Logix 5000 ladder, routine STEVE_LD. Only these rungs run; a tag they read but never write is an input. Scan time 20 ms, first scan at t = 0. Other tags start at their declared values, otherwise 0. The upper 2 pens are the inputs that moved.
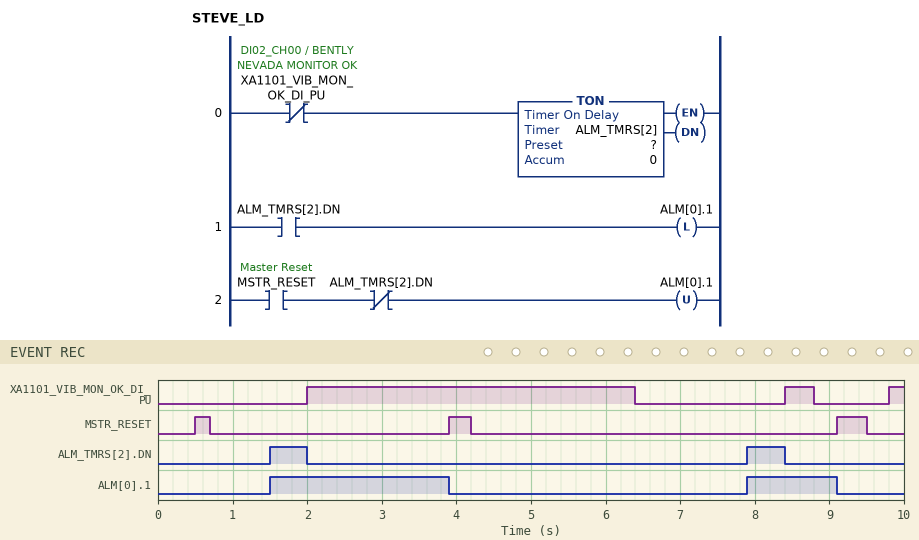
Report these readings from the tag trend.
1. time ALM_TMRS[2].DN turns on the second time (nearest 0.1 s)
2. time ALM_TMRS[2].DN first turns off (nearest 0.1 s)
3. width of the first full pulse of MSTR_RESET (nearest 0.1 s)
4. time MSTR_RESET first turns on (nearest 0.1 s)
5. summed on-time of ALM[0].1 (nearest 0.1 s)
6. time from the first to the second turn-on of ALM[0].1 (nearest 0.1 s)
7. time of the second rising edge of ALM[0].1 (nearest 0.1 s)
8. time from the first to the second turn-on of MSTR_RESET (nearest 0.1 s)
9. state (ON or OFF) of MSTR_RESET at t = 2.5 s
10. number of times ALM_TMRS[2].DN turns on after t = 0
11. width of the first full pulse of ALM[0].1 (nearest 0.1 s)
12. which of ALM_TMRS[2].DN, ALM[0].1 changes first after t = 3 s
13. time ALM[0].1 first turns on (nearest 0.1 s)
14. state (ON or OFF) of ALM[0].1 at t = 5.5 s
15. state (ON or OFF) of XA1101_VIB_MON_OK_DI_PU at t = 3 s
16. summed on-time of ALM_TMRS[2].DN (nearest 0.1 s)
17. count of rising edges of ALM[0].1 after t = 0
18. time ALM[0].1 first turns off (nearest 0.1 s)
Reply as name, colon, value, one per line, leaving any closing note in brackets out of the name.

time ALM_TMRS[2].DN turns on the second time: 7.9 s
time ALM_TMRS[2].DN first turns off: 2.0 s
width of the first full pulse of MSTR_RESET: 0.2 s
time MSTR_RESET first turns on: 0.5 s
summed on-time of ALM[0].1: 3.6 s
time from the first to the second turn-on of ALM[0].1: 6.4 s
time of the second rising edge of ALM[0].1: 7.9 s
time from the first to the second turn-on of MSTR_RESET: 3.4 s
state (ON or OFF) of MSTR_RESET at t = 2.5 s: OFF
number of times ALM_TMRS[2].DN turns on after t = 0: 2
width of the first full pulse of ALM[0].1: 2.4 s
which of ALM_TMRS[2].DN, ALM[0].1 changes first after t = 3 s: ALM[0].1
time ALM[0].1 first turns on: 1.5 s
state (ON or OFF) of ALM[0].1 at t = 5.5 s: OFF
state (ON or OFF) of XA1101_VIB_MON_OK_DI_PU at t = 3 s: ON
summed on-time of ALM_TMRS[2].DN: 1.0 s
count of rising edges of ALM[0].1 after t = 0: 2
time ALM[0].1 first turns off: 3.9 s
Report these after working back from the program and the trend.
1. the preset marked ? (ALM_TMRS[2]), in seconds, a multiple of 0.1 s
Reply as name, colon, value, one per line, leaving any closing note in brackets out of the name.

the preset marked ? (ALM_TMRS[2]), in seconds, a multiple of 0.1 s: 1.5 s
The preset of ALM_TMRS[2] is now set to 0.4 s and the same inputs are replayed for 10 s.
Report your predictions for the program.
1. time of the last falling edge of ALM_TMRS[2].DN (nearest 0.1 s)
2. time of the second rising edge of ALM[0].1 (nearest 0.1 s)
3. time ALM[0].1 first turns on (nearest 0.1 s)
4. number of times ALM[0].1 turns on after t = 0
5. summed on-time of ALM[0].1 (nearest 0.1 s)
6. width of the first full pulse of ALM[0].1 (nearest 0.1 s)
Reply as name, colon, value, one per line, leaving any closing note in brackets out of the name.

time of the last falling edge of ALM_TMRS[2].DN: 9.8 s
time of the second rising edge of ALM[0].1: 6.8 s
time ALM[0].1 first turns on: 0.4 s
number of times ALM[0].1 turns on after t = 0: 3
summed on-time of ALM[0].1: 6.6 s
width of the first full pulse of ALM[0].1: 3.5 s
